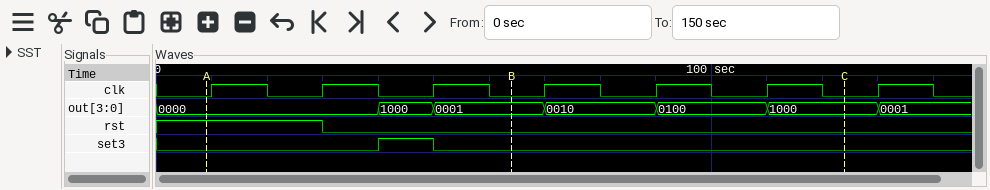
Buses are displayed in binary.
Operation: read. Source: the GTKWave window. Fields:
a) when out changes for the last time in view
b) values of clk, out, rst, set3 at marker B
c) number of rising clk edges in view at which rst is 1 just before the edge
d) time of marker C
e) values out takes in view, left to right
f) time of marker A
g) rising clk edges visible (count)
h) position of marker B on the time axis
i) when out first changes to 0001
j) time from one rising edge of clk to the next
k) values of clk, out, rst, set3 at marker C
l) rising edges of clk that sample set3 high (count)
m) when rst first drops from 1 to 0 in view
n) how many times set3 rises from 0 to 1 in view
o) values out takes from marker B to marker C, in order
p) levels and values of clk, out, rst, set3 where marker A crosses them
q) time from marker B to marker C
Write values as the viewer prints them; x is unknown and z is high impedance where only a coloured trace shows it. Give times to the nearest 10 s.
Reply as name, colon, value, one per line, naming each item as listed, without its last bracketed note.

when out changes for the last time in view: 130 s
values of clk, out, rst, set3 at marker B: clk=0, out=0001, rst=0, set3=0
number of rising clk edges in view at which rst is 1 just before the edge: 2
time of marker C: 120 s
values out takes in view, left to right: 0000, 1000, 0001, 0010, 0100, 1000, 0001
time of marker A: 10 s
rising clk edges visible: 7
position of marker B on the time axis: 60 s
when out first changes to 0001: 50 s
time from one rising edge of clk to the next: 20 s
values of clk, out, rst, set3 at marker C: clk=0, out=1000, rst=0, set3=0
rising edges of clk that sample set3 high: 1
when rst first drops from 1 to 0 in view: 30 s
how many times set3 rises from 0 to 1 in view: 1
values out takes from marker B to marker C, in order: 0001, 0010, 0100, 1000
levels and values of clk, out, rst, set3 where marker A crosses them: clk=0, out=0000, rst=1, set3=0
time from marker B to marker C: 60 s
